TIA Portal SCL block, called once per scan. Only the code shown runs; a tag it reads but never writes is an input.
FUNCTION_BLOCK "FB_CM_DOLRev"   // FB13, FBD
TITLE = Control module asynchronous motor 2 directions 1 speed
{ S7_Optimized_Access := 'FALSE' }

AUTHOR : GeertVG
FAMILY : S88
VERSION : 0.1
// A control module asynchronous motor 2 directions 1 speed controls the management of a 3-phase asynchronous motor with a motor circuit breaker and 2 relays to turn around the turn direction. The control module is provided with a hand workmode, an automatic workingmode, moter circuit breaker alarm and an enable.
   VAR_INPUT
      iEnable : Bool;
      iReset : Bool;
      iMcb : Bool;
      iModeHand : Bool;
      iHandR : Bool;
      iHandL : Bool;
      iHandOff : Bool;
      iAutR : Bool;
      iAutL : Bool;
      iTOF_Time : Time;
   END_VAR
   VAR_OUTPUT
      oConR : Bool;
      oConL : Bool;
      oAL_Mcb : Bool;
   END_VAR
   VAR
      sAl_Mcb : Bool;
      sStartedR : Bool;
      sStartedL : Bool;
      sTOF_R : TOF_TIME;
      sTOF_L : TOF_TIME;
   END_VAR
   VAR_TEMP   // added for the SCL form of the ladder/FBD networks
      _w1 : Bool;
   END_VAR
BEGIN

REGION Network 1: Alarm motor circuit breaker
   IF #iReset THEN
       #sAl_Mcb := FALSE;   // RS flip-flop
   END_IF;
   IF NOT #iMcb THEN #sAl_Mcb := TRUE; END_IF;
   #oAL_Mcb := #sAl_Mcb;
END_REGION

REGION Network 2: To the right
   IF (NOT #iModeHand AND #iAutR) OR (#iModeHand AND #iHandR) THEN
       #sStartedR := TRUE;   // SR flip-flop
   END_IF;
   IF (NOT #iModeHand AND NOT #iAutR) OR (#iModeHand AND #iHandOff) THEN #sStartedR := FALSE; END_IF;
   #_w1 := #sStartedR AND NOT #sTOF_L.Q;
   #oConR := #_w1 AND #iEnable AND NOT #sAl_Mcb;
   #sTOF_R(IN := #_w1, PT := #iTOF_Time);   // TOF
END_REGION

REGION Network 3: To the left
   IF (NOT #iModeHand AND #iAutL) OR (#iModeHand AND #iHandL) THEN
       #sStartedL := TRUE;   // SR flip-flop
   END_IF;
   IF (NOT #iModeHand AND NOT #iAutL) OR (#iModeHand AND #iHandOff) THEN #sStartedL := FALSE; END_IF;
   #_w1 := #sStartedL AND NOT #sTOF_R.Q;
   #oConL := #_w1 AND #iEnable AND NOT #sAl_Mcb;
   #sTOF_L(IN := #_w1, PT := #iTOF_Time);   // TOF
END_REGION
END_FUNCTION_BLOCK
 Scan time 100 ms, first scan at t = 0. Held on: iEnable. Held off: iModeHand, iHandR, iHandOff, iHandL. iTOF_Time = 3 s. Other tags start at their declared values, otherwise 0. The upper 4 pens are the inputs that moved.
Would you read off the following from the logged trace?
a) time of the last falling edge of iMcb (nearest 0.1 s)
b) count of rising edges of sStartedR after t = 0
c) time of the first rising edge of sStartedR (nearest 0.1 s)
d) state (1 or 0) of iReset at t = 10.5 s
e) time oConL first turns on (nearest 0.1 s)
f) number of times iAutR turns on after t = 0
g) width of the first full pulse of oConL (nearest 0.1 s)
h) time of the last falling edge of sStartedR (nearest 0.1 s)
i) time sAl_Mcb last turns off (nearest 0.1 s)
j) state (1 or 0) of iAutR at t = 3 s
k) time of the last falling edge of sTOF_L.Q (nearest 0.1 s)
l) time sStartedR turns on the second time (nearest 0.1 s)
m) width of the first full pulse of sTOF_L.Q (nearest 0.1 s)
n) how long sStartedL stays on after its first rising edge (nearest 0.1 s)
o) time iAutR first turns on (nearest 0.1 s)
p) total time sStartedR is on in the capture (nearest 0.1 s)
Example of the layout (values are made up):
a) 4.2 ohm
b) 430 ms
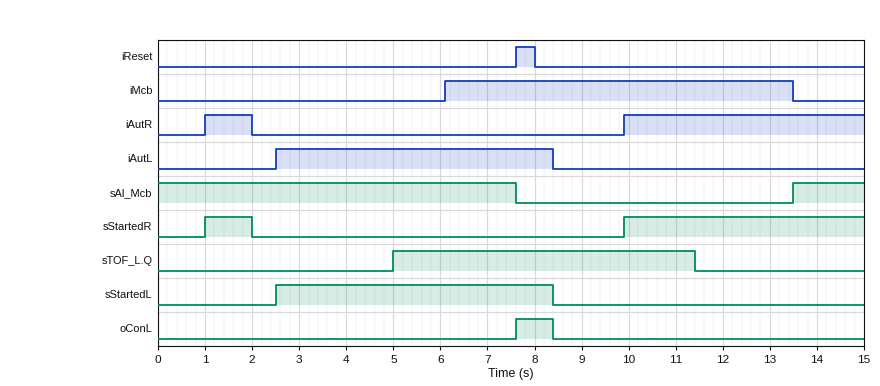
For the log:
a) 13.5 s
b) 2
c) 1.0 s
d) 0
e) 7.6 s
f) 2
g) 0.8 s
h) 2.0 s
i) 7.6 s
j) 0
k) 11.4 s
l) 9.9 s
m) 6.4 s
n) 5.9 s
o) 1.0 s
p) 6.1 s
